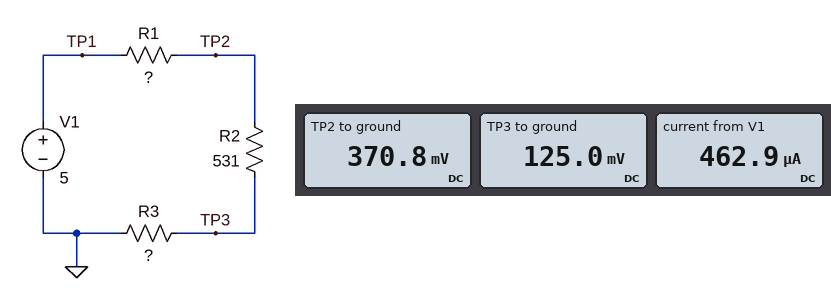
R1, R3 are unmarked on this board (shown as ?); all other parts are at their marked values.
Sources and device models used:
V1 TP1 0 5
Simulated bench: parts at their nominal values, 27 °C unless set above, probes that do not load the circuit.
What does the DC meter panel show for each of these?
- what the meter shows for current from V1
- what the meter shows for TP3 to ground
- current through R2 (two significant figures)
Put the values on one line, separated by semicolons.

462.9 µA; 125.0 mV; 460 µA
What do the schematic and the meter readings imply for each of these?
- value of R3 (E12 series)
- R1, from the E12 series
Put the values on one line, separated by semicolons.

270 Ω; 10 kΩ
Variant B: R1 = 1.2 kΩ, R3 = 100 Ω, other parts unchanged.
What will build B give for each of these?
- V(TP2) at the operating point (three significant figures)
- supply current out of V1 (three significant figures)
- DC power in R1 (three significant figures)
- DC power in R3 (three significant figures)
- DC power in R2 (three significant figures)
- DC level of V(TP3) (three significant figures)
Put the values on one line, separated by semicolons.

1.72 V; 2.73 mA; 8.95 mW; 746 µW; 3.96 mW; 273 mV
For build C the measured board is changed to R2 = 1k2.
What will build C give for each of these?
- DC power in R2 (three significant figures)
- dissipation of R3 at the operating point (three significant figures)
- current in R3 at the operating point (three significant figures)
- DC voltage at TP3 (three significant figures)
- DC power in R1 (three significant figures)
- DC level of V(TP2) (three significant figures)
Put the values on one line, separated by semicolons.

228 µW; 51.3 µW; 436 µA; 118 mV; 1.90 mW; 641 mV
